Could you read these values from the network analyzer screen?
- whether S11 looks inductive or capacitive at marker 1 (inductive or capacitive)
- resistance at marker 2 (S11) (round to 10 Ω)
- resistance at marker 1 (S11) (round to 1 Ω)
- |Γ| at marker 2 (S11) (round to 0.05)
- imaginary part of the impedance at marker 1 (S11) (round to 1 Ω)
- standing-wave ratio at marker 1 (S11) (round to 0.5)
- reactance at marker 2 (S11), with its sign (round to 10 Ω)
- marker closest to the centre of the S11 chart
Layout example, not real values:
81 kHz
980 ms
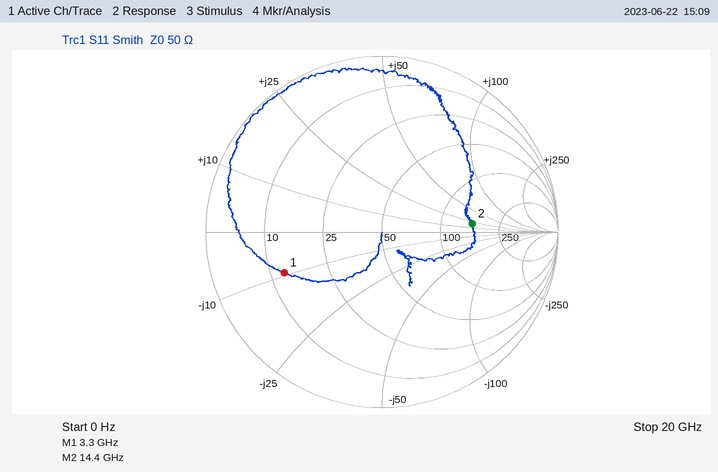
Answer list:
capacitive
150 Ω
13 Ω
0.50
-9 Ω
4.0
+20 Ω
marker 2
